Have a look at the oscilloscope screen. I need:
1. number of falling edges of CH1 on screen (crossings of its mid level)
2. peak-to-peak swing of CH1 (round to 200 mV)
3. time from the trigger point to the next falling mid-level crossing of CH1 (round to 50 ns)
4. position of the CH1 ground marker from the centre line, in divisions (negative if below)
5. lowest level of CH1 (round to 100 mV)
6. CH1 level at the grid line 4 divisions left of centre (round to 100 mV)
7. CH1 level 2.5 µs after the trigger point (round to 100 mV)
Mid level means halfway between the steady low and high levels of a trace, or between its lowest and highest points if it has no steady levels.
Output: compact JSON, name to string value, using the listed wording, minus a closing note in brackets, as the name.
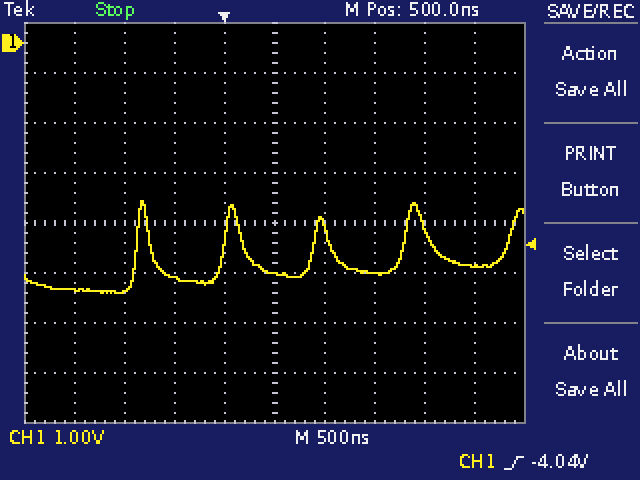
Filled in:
{"number of falling edges of CH1 on screen": "4", "peak-to-peak swing of CH1": "1.8 V", "time from the trigger point to the next falling mid-level crossing of CH1": "200 ns", "position of the CH1 ground marker from the centre line, in divisions": "+3.6 div", "lowest level of CH1": "-5.0 V", "CH1 level at the grid line 4 divisions left of centre": "-4.9 V", "CH1 level 2.5 µs after the trigger point": "-4.5 V"}
